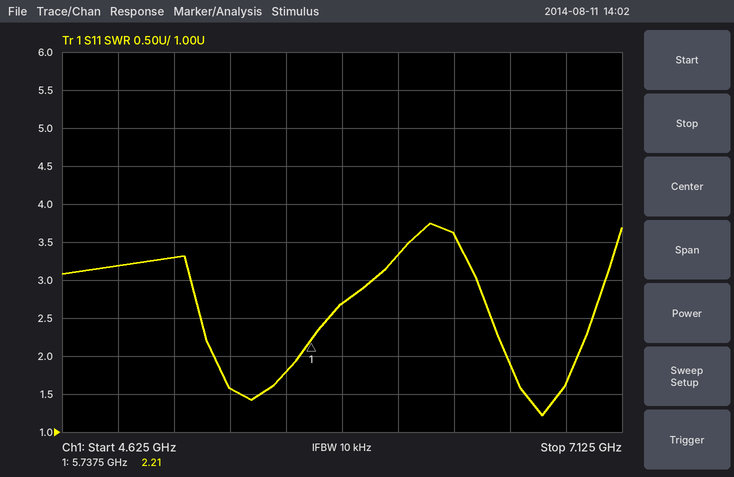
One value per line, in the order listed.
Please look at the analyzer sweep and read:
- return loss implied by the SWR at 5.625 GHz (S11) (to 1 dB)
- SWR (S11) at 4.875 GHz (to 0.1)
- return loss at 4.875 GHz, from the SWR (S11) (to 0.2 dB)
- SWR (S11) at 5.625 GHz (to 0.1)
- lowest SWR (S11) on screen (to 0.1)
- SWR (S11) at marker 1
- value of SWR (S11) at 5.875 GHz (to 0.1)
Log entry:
11 dB
3.2
5.6 dB
1.8
1.2
2.21
2.7
